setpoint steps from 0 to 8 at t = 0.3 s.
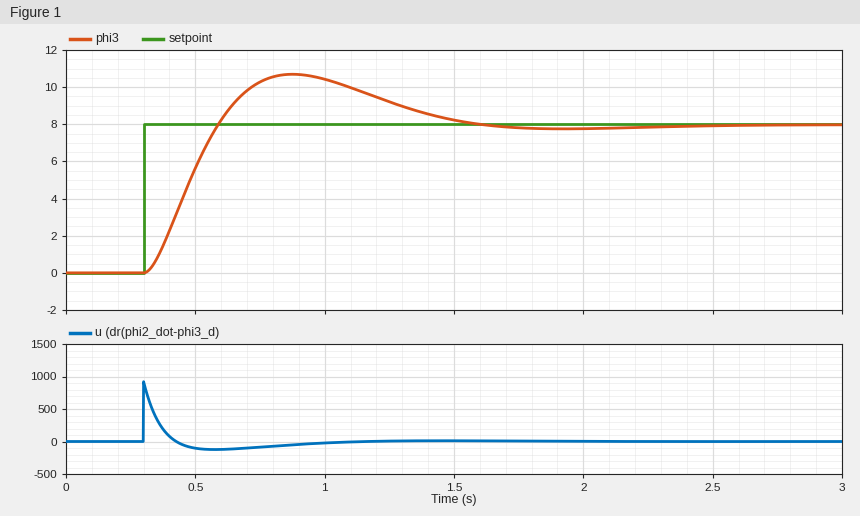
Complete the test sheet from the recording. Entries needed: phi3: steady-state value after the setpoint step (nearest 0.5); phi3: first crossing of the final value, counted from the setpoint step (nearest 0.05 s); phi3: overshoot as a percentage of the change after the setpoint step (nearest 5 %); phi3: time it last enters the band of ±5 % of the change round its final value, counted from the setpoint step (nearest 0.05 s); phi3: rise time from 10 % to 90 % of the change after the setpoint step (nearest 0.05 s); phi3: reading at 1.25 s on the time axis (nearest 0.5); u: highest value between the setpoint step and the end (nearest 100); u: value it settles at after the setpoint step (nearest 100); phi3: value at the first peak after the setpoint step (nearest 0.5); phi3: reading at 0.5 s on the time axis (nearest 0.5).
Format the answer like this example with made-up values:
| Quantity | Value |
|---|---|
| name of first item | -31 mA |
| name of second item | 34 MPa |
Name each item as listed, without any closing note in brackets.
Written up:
| Quantity | Value |
|---|---|
| phi3: steady-state value after the setpoint step | 8.0 |
| phi3: first crossing of the final value, counted from the setpoint step | 0.30 s |
| phi3: overshoot as a percentage of the change after the setpoint step | 35 % |
| phi3: time it last enters the band of ±5 % of the change round its final value, counted from the setpoint step | 1.15 s |
| phi3: rise time from 10 % to 90 % of the change after the setpoint step | 0.20 s |
| phi3: reading at 1.25 s on the time axis | 9.0 |
| u: highest value between the setpoint step and the end | 900 |
| u: value it settles at after the setpoint step | 0 |
| phi3: value at the first peak after the setpoint step | 10.5 |
| phi3: reading at 0.5 s on the time axis | 5.5 |
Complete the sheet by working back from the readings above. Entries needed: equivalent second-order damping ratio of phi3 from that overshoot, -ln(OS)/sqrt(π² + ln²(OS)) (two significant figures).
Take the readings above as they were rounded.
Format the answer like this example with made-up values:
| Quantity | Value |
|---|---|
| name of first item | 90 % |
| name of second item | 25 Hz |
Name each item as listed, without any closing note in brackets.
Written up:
| Quantity | Value |
|---|---|
| equivalent second-order damping ratio of phi3 from that overshoot, -ln(OS)/sqrt(π² + ln²(OS)) | 0.32 |
